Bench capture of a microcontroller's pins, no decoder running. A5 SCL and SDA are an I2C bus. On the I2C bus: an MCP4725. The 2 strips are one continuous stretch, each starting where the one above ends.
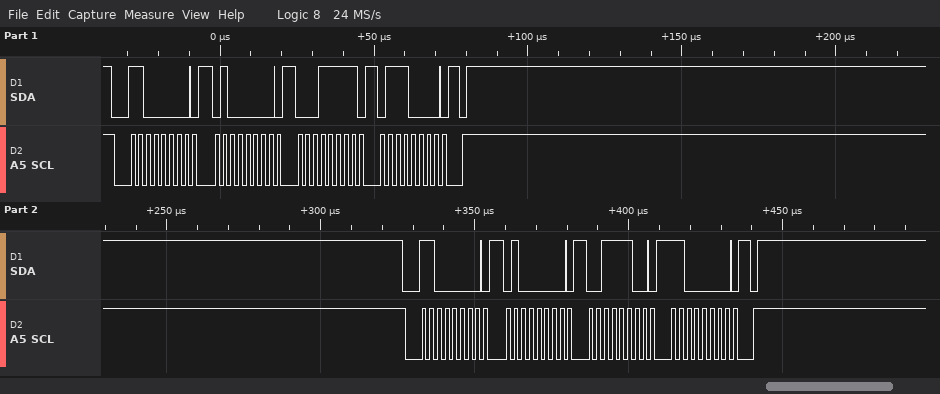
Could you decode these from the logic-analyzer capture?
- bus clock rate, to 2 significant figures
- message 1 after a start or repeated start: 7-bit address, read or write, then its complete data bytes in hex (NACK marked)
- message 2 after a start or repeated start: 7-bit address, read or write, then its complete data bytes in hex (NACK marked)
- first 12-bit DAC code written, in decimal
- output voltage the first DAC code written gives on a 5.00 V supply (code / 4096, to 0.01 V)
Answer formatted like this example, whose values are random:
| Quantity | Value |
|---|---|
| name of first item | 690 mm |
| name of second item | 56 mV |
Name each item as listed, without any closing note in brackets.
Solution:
| Quantity | Value |
|---|---|
| bus clock rate, to 2 significant figures | 400 kHz |
| message 1 after a start or repeated start: 7-bit address, read or write, then its complete data bytes in hex | 0x60 write: 40 1F 70 |
| message 2 after a start or repeated start: 7-bit address, read or write, then its complete data bytes in hex | 0x60 write: 40 3C C0 |
| first 12-bit DAC code written, in decimal | 503 |
| output voltage the first DAC code written gives on a 5.00 V supply | 0.61 V |
